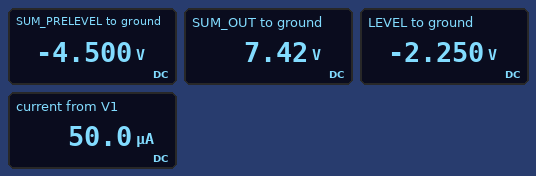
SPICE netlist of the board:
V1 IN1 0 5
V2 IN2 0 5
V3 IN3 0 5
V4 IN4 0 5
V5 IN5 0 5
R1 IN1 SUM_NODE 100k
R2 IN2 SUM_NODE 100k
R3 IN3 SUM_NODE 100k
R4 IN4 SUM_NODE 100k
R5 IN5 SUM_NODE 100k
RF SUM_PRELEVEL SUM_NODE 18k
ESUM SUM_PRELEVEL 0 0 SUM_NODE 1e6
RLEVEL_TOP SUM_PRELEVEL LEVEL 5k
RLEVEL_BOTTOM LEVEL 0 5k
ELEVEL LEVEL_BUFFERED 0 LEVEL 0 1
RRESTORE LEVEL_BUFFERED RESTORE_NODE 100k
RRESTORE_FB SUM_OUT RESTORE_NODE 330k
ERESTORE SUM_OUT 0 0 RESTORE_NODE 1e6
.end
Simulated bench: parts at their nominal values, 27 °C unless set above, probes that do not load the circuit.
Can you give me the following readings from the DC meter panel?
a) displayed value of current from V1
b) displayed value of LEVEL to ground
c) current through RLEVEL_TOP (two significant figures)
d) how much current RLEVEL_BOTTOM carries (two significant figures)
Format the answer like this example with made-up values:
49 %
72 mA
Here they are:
50.0 µA
-2.250 V
450 µA
450 µA
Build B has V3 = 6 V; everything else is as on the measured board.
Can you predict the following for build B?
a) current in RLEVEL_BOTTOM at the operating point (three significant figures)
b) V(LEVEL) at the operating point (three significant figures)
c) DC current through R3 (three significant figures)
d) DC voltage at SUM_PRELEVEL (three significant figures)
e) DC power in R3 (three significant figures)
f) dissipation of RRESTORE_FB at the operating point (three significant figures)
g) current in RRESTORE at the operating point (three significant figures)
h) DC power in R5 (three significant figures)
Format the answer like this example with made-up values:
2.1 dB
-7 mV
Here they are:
468 µA
-2.34 V
60.0 µA
-4.68 V
360 µW
181 µW
23.4 µA
250 µW
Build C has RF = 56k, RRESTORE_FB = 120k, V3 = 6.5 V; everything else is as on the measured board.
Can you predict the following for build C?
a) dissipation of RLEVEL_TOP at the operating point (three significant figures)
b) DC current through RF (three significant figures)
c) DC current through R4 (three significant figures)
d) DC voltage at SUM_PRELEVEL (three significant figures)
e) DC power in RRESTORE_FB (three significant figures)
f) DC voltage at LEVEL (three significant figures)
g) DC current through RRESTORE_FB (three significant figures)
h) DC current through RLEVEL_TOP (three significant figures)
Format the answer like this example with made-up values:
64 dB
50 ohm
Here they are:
11.0 mW
265 µA
50.0 µA
-14.8 V
661 µW
-7.42 V
74.2 µA
1.48 mA
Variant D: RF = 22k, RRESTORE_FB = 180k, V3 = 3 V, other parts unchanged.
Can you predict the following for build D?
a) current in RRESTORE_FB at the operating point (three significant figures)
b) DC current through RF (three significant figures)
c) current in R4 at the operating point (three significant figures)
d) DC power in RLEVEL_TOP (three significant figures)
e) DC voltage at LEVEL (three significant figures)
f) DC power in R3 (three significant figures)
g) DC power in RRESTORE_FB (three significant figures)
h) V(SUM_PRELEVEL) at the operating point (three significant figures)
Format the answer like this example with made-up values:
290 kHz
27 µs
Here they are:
25.3 µA
230 µA
50.0 µA
1.28 mW
-2.53 V
90.0 µW
115 µW
-5.06 V
